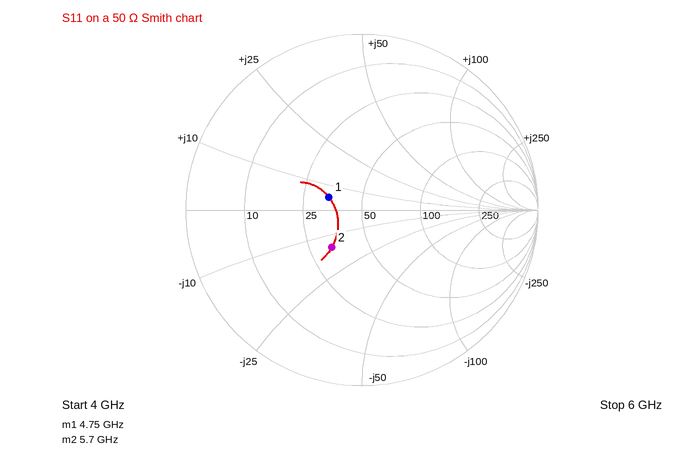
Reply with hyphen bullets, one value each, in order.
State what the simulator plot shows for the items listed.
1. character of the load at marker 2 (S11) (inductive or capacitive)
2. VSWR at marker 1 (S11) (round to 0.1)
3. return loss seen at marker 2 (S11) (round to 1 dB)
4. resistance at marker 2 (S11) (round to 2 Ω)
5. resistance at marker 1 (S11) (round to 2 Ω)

- capacitive
- 1.5
- 11 dB
- 32 Ω
- 34 Ω
